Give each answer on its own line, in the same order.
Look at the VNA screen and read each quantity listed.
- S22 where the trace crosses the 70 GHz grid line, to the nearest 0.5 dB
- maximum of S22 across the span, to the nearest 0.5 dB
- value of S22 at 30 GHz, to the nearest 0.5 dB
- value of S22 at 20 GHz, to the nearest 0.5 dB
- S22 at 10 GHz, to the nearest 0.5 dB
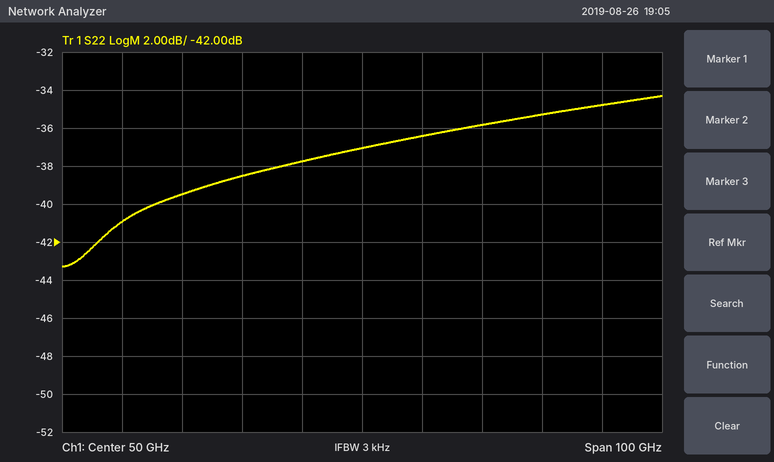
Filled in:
-36.0 dB
-34.5 dB
-38.5 dB
-39.5 dB
-41.0 dB
